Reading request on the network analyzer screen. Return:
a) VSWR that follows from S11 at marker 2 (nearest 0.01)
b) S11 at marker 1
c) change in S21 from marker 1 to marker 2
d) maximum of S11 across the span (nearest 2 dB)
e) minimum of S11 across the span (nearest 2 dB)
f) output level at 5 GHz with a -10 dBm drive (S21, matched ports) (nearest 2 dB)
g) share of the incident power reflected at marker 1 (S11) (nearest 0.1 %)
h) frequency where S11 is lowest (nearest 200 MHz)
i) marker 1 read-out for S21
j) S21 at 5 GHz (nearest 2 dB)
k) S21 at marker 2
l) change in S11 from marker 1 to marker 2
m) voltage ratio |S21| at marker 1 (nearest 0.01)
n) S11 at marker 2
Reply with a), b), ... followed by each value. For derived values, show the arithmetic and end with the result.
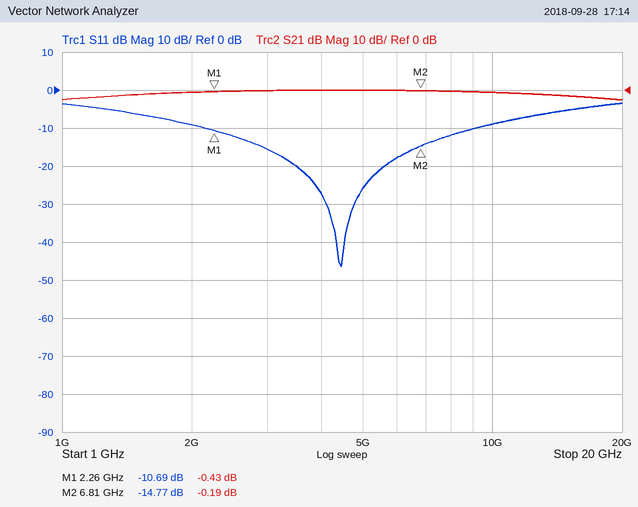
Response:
a) (1 + 0.1826)/(1 − 0.1826) ≈ 1.45
b) -10.69 dB
c) -0.19 − (-0.43) = 0.24 dB
d) -4 dB
e) -46 dB
f) -10 dBm + (0 dB) = -10 dBm
g) 10^(-10.69/10) ≈ 8.5 %
h) 4.4 GHz
i) -0.43 dB
j) 0 dB
k) -0.19 dB
l) -14.77 − (-10.69) = -4.08 dB
m) 10^(-0.43/20) ≈ 0.95
n) -14.77 dB
